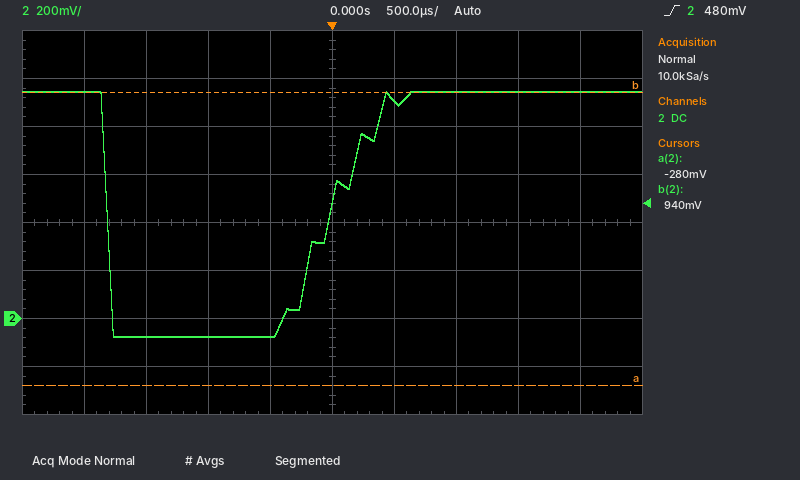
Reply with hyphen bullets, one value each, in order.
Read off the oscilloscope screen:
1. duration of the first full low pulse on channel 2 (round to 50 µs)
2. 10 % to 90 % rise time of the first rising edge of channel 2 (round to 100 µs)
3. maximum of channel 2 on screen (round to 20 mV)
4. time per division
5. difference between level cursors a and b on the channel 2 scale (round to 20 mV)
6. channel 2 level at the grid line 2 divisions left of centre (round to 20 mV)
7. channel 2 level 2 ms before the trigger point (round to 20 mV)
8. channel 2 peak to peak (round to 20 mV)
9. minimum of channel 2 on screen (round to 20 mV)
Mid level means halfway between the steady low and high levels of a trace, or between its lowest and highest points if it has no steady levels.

- 1.80 ms
- 800 µs
- 940 mV
- 500 µs
- 1.22 V
- -80 mV
- 940 mV
- 1.02 V
- -80 mV
